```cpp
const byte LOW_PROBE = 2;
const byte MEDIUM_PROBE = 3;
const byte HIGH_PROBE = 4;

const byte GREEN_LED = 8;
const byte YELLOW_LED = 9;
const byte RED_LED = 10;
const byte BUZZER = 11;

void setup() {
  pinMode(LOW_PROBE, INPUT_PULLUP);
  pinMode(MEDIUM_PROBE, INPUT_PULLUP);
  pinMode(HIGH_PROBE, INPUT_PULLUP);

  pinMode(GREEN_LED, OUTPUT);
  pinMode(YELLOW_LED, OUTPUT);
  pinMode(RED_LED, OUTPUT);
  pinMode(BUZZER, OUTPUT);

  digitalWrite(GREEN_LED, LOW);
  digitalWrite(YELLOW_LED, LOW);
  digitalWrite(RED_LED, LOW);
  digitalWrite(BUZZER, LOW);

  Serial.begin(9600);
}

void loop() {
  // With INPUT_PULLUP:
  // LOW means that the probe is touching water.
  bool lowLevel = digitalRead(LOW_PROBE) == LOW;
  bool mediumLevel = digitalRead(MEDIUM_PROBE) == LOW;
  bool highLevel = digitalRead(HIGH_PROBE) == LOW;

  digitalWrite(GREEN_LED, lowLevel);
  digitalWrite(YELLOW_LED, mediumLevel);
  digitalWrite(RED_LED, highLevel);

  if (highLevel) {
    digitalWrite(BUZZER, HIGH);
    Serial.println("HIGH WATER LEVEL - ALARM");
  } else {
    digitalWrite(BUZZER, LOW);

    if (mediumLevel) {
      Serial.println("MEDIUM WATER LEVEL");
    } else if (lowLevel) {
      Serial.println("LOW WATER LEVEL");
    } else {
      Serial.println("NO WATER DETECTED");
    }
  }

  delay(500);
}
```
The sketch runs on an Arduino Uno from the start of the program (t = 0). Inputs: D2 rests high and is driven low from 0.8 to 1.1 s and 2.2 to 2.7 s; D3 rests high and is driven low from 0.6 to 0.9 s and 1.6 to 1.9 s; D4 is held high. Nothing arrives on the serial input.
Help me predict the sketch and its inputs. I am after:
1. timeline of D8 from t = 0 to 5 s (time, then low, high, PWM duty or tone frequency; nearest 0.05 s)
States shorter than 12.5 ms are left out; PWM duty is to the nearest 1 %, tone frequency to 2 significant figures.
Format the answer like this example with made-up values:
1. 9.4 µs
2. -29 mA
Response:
1. 0 s low; 1 s high; 1.5 s low; 2.5 s high; 3 s low
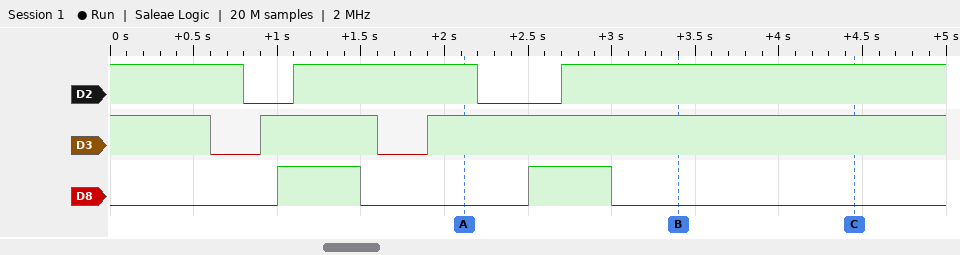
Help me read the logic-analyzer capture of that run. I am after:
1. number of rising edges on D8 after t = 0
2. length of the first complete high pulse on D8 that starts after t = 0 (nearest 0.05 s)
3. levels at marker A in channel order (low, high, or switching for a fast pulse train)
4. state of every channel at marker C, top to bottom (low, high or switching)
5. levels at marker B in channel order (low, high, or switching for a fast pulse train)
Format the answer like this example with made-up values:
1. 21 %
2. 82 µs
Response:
1. 2
2. 0.50 s
3. D2 high, D3 high, D8 low
4. D2 high, D3 high, D8 low
5. D2 high, D3 high, D8 low
